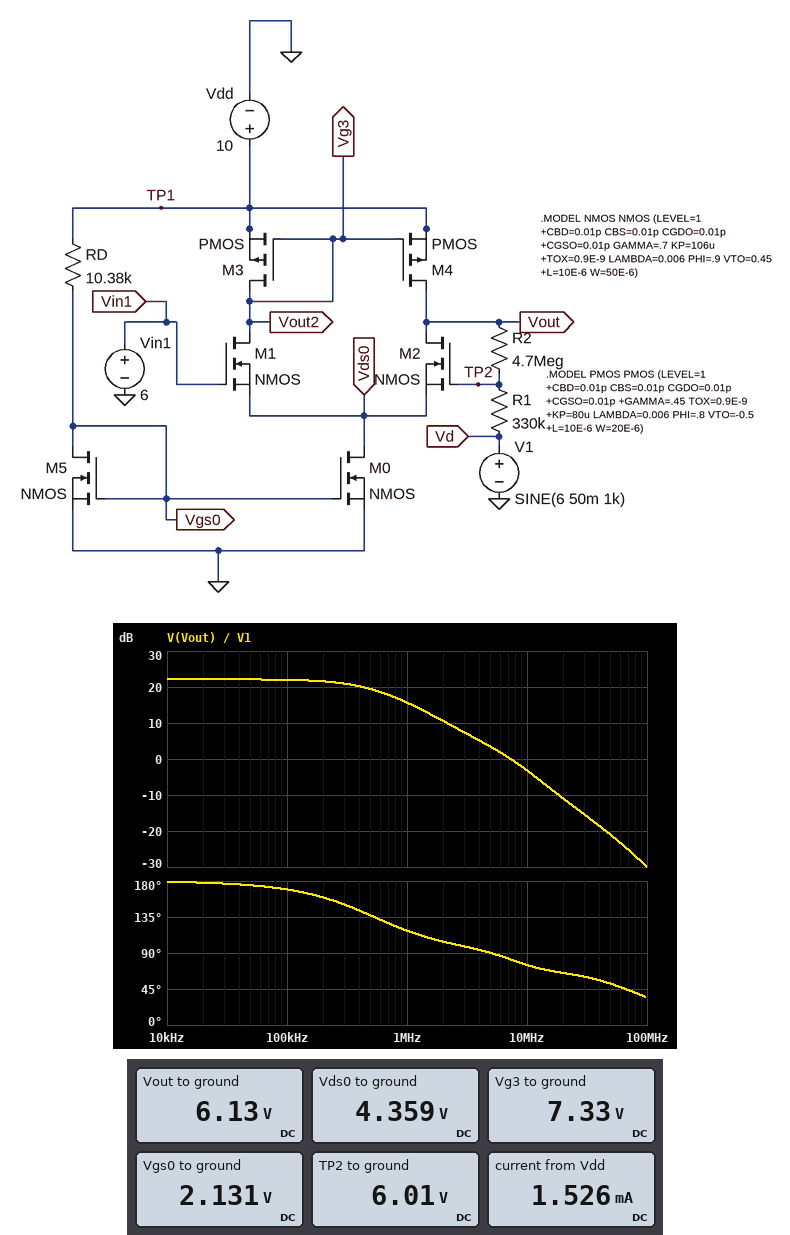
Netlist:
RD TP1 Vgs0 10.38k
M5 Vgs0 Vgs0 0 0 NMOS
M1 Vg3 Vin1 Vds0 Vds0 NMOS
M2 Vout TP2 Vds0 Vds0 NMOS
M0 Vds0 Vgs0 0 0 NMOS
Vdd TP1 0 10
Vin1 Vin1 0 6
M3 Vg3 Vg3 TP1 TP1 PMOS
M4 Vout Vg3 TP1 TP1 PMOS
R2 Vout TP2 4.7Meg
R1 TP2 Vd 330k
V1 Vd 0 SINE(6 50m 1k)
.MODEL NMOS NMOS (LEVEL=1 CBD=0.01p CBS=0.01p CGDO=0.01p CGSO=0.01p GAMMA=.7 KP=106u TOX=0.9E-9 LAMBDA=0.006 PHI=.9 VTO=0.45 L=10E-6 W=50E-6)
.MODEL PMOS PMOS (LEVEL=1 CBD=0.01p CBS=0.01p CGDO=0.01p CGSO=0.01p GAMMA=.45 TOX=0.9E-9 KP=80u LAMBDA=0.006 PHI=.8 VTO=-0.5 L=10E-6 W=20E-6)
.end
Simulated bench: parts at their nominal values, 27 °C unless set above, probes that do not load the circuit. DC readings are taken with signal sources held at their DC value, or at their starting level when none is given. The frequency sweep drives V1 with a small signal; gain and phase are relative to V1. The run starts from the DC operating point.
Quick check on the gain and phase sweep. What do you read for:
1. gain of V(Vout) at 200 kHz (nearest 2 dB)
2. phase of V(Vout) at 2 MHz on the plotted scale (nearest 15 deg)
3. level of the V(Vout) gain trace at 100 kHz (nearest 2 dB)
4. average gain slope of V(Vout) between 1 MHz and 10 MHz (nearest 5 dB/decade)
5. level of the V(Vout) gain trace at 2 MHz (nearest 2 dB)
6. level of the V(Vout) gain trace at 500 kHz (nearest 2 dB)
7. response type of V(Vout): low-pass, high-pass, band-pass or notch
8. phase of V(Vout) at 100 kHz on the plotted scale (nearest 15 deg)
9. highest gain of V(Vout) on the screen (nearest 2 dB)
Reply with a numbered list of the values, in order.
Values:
1. 22 dB
2. 105 deg
3. 22 dB
4. -20 dB/decade
5. 10 dB
6. 20 dB
7. low-pass
8. 165 deg
9. 22 dB
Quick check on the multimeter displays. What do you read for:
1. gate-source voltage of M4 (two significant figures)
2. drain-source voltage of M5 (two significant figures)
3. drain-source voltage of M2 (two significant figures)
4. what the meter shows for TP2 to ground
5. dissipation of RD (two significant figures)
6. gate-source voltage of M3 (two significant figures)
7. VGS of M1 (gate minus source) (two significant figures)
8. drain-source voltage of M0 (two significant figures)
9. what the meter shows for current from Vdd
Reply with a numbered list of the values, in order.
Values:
1. -2.7 V
2. 2.1 V
3. 1.8 V
4. 6.01 V
5. 6.0 mW
6. -2.7 V
7. 1.6 V
8. 4.4 V
9. 1.526 mA
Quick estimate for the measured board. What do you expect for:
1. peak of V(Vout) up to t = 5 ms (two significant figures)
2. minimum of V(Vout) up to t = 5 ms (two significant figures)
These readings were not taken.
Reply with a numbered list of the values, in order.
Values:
1. 6.8 V
2. 5.5 V
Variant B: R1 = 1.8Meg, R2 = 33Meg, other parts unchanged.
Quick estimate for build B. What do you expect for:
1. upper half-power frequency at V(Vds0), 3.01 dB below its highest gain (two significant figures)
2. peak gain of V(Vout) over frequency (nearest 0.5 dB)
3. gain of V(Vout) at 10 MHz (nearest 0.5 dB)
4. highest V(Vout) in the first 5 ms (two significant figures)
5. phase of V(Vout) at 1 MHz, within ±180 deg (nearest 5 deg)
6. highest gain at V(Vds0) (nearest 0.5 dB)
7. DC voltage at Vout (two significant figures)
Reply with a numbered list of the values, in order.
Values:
1. 80 kHz
2. 24.0 dB
3. -17.5 dB
4. 7.0 V
5. 95 deg
6. -31.0 dB
7. 6.2 V
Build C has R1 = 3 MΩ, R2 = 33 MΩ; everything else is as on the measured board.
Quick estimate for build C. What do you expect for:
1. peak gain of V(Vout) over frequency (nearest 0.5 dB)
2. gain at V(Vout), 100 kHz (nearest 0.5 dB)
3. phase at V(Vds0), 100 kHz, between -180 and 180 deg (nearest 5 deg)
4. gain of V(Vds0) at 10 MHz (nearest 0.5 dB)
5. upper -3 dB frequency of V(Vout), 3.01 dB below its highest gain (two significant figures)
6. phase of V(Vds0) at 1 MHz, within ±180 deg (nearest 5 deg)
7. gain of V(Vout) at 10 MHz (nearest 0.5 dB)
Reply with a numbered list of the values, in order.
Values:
1. 20.0 dB
2. 16.0 dB
3. -50 deg
4. -69.0 dB
5. 76 kHz
6. -75 deg
7. -22.0 dB
